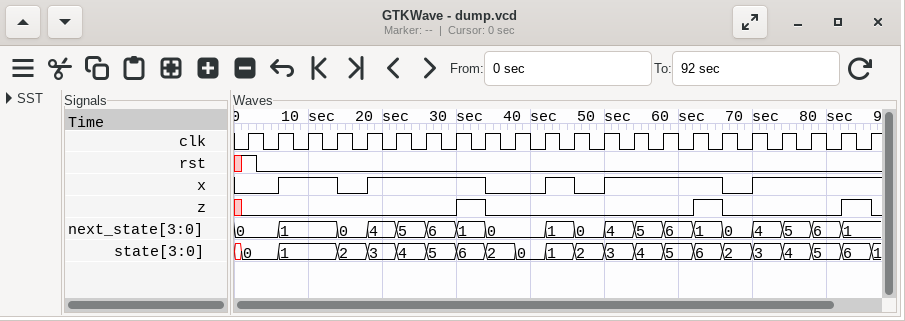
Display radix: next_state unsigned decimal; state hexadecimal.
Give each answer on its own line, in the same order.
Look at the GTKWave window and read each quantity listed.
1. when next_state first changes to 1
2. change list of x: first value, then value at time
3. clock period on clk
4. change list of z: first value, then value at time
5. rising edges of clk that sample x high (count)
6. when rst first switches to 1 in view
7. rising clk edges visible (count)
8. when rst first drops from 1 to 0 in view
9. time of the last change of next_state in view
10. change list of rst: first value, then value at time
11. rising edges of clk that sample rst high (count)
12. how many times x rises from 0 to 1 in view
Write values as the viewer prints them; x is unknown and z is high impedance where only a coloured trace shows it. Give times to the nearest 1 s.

6 s
0, 1 at 6 s, 0 at 14 s, 1 at 18 s, 0 at 34 s, 1 at 42 s, 0 at 46 s, 1 at 50 s, 0 at 66 s, 1 at 70 s
4 s
x, 0 at 1 s, 1 at 30 s, 0 at 34 s, 1 at 62 s, 0 at 66 s, 1 at 82 s, 0 at 86 s
15
1 s
22
3 s
82 s
x, 1 at 1 s, 0 at 3 s
1
5
